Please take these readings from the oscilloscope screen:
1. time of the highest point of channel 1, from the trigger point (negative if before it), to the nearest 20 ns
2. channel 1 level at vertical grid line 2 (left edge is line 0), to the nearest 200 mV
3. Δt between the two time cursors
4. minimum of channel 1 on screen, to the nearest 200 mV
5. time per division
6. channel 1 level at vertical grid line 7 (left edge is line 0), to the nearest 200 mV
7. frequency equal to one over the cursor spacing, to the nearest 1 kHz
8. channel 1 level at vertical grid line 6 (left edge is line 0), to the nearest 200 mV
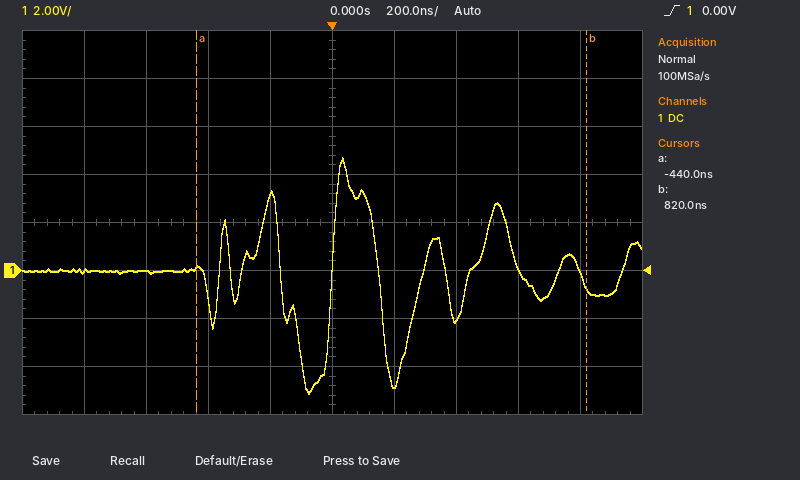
+40 ns
0.0 V
1.26 µs
-5.2 V
200 ns
-2.0 V
794 kHz
-4.8 V
